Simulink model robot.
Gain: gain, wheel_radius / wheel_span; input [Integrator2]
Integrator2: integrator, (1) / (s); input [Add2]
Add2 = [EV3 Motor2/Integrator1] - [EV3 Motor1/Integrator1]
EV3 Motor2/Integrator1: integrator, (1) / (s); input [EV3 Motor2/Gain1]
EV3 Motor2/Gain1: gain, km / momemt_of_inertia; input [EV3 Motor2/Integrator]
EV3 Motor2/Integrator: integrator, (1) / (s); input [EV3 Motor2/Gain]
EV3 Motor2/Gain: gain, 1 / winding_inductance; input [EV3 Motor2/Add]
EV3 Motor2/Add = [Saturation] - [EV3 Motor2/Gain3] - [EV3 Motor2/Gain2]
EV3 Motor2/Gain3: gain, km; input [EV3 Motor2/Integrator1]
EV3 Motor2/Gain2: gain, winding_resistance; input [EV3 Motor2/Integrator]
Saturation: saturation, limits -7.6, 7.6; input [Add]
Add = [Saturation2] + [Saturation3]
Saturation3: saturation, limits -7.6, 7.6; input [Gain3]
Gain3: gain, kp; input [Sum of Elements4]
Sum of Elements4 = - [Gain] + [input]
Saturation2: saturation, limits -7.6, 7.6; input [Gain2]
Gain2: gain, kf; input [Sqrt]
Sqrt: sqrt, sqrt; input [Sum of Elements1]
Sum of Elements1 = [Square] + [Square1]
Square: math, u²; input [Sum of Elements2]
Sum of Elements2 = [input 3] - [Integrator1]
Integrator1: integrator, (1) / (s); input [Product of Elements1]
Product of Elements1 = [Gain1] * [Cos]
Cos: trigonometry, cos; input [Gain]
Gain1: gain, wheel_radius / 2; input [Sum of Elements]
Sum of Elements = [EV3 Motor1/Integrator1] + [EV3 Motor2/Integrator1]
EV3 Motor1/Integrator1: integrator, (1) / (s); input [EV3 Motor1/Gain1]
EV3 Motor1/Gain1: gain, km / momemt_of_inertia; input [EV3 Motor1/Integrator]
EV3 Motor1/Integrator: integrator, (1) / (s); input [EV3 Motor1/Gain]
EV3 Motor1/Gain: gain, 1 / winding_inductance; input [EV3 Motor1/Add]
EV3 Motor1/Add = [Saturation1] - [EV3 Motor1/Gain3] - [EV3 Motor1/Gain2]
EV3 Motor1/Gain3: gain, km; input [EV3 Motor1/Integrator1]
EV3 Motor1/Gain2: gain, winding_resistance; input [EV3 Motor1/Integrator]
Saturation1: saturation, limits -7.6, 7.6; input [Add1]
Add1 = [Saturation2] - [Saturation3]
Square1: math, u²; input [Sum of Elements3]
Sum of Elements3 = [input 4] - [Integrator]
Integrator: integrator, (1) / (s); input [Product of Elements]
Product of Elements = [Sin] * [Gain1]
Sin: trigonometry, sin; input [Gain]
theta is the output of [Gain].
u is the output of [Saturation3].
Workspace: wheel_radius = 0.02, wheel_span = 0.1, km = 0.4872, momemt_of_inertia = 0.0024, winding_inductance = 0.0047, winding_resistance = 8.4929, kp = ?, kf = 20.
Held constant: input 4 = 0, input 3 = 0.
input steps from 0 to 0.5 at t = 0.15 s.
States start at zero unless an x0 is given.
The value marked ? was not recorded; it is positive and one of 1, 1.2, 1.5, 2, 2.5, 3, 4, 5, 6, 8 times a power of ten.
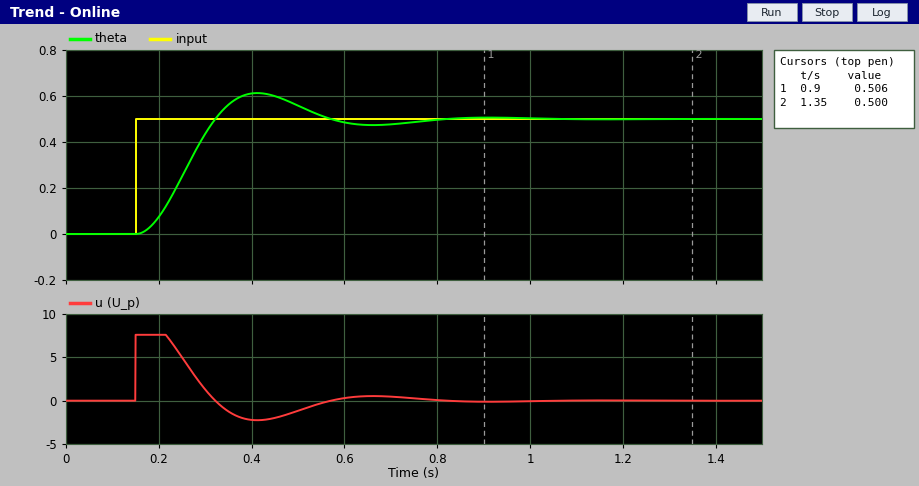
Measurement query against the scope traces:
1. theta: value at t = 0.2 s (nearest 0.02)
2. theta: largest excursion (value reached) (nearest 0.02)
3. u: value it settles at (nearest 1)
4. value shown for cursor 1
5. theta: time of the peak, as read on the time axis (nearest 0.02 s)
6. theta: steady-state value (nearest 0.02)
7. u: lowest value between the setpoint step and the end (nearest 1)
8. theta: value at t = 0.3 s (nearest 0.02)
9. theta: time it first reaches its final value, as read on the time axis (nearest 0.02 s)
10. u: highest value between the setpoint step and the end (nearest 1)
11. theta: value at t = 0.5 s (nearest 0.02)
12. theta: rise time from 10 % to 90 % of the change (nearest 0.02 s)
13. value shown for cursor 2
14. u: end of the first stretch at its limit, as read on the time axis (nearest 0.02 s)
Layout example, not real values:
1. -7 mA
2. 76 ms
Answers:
1. 0.08
2. 0.62
3. 0
4. 0.506
5. 0.42 s
6. 0.50
7. -2
8. 0.44
9. 0.32 s
10. 8
11. 0.56
12. 0.12 s
13. 0.500
14. 0.22 s
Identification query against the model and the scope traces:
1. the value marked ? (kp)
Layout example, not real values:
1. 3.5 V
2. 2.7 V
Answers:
1. 20
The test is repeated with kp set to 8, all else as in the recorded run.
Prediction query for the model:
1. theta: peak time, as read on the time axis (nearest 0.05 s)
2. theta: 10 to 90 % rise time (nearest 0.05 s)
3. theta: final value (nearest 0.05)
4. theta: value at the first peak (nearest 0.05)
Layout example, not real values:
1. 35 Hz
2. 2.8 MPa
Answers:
1. 0.65 s
2. 0.25 s
3. 0.50
4. 0.55
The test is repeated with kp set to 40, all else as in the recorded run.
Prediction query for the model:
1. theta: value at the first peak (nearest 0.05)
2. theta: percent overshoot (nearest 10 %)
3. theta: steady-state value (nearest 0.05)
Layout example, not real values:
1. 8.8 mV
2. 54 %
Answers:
1. 0.65
2. 30 %
3. 0.50
